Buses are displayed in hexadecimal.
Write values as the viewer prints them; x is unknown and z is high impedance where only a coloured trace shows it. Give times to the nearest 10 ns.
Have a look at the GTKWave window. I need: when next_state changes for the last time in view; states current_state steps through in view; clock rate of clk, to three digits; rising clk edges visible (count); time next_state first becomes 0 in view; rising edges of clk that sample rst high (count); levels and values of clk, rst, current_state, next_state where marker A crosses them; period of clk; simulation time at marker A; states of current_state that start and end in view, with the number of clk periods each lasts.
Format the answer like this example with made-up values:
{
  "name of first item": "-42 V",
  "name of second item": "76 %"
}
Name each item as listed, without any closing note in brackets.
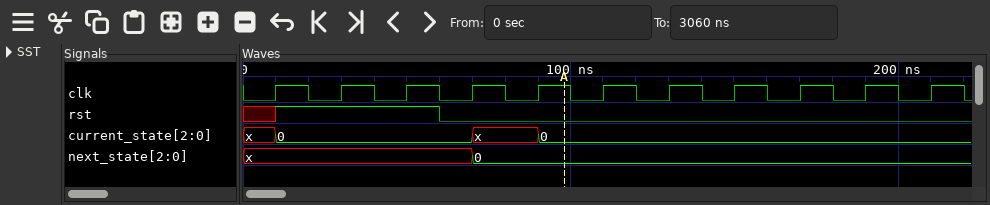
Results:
{
  "when next_state changes for the last time in view": "70 ns",
  "states current_state steps through in view": "x, 0, x, 0",
  "clock rate of clk, to three digits": "50.0 MHz",
  "rising clk edges visible": "11",
  "time next_state first becomes 0 in view": "70 ns",
  "rising edges of clk that sample rst high": "2",
  "levels and values of clk, rst, current_state, next_state where marker A crosses them": "clk=1, rst=0, current_state=0, next_state=0",
  "period of clk": "20 ns",
  "simulation time at marker A": "100 ns",
  "states of current_state that start and end in view, with the number of clk periods each lasts": "0: 3, x: 1"
}
